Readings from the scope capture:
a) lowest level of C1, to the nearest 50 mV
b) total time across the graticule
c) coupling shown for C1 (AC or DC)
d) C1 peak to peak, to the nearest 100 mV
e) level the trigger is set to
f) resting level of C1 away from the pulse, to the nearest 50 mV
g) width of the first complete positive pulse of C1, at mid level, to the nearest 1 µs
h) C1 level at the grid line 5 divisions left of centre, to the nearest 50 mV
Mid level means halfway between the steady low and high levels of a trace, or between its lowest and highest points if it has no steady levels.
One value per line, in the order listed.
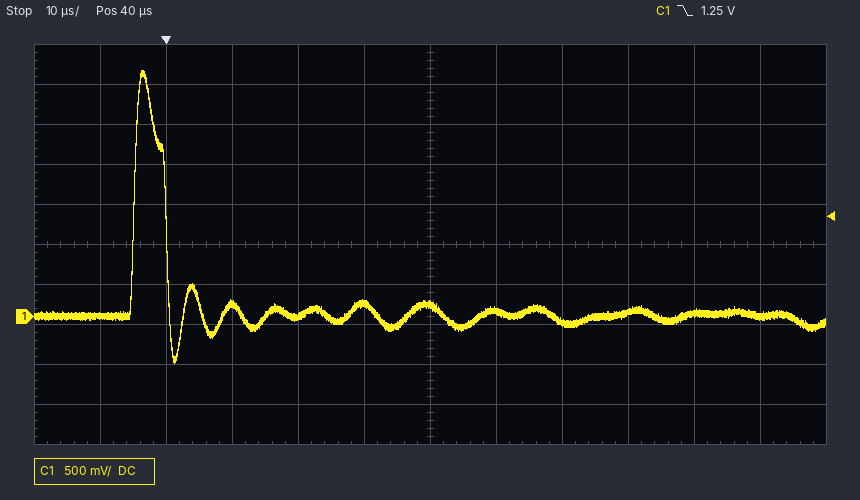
-600 mV
120 µs
DC
3.70 V
1.25 V
0 mV
5 µs
0 mV
